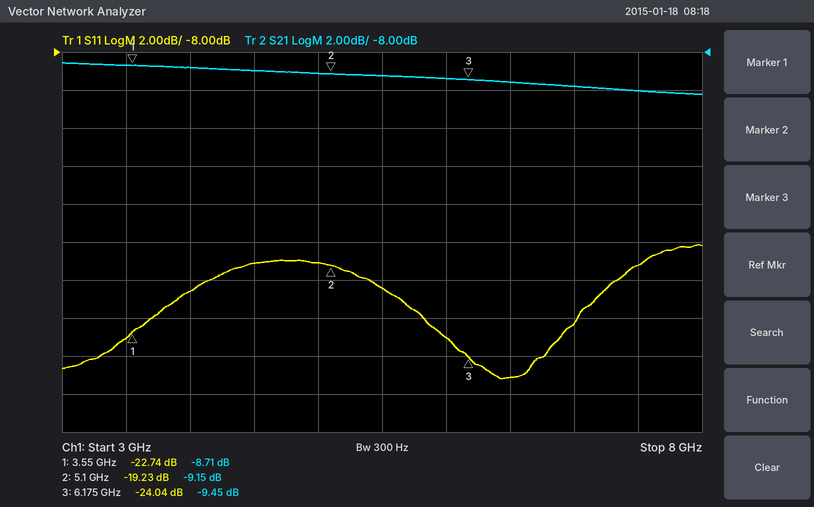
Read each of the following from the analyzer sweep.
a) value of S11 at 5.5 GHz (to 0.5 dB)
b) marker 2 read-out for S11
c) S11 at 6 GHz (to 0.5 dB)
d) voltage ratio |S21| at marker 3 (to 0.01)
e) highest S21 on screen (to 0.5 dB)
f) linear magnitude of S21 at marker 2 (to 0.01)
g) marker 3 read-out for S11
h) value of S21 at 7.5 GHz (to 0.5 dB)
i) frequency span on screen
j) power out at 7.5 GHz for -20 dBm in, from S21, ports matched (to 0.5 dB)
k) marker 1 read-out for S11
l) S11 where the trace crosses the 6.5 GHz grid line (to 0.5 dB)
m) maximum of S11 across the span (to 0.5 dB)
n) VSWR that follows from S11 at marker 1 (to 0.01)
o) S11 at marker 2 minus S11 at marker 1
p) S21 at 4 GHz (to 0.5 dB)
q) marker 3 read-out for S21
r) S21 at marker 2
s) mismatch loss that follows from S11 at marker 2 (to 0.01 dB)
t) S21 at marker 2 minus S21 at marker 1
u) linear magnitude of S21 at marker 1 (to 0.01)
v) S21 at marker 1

-20.5 dB
-19.23 dB
-23.0 dB
0.34
-8.5 dB
0.35
-24.04 dB
-10.0 dB
5 GHz
-30.0 dBm
-22.74 dB
-25.0 dB
-18.0 dB
1.16
3.51 dB
-9.0 dB
-9.45 dB
-9.15 dB
0.05 dB
-0.44 dB
0.37
-8.71 dB
